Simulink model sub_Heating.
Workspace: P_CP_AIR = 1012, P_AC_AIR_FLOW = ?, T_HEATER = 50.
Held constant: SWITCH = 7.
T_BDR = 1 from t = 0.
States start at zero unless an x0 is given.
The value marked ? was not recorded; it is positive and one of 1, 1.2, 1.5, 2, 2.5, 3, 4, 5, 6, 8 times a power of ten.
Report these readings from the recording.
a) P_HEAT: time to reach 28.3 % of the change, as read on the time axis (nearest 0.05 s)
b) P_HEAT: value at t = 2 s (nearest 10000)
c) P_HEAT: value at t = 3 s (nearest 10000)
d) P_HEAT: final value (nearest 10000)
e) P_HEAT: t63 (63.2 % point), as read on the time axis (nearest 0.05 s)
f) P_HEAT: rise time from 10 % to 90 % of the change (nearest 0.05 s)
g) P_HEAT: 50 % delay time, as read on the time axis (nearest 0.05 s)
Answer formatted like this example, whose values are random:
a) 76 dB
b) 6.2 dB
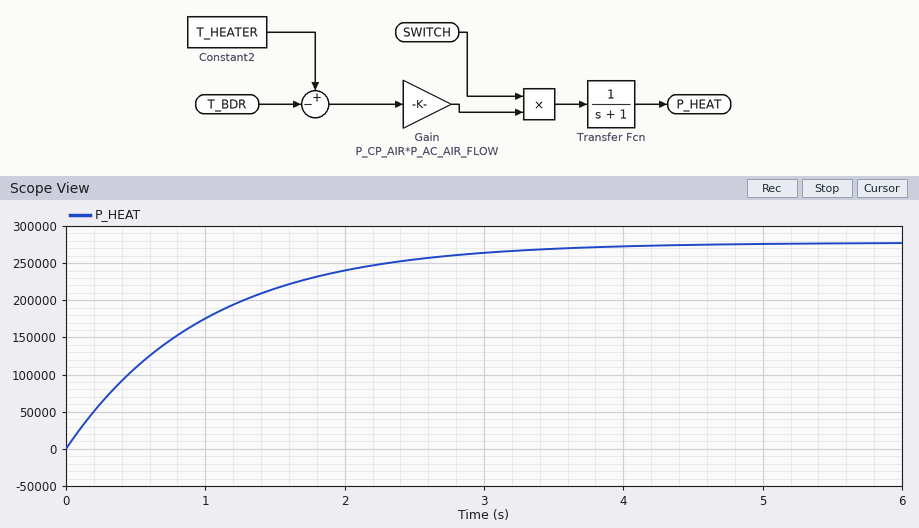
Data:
a) 0.35 s
b) 240000
c) 260000
d) 280000
e) 1.00 s
f) 2.20 s
g) 0.70 s
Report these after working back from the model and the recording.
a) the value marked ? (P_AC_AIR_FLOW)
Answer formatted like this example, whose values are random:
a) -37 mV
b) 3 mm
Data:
a) 0.8
